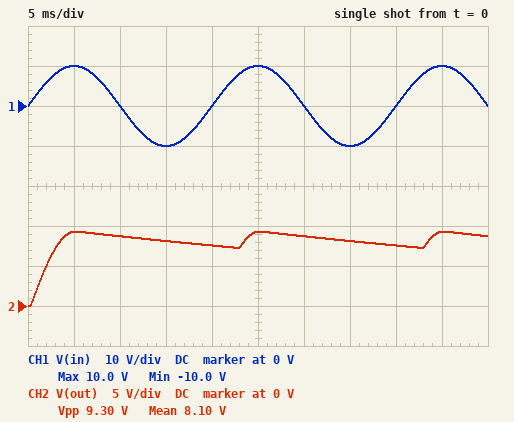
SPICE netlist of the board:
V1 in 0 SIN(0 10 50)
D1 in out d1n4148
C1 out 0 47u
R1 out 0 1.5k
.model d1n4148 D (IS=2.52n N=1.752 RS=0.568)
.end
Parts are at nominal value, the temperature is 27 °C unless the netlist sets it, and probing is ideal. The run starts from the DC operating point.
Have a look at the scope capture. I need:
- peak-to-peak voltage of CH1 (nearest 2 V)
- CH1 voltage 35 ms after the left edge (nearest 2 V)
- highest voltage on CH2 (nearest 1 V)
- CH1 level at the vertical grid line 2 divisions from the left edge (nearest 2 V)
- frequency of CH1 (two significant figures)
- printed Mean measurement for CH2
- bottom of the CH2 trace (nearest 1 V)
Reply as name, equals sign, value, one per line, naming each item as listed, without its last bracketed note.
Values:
peak-to-peak voltage of CH1 = 20 V
CH1 voltage 35 ms after the left edge = -10 V
highest voltage on CH2 = 9 V
CH1 level at the vertical grid line 2 divisions from the left edge = 0 V
frequency of CH1 = 50 Hz
printed Mean measurement for CH2 = 8.10 V
bottom of the CH2 trace = 0 V
